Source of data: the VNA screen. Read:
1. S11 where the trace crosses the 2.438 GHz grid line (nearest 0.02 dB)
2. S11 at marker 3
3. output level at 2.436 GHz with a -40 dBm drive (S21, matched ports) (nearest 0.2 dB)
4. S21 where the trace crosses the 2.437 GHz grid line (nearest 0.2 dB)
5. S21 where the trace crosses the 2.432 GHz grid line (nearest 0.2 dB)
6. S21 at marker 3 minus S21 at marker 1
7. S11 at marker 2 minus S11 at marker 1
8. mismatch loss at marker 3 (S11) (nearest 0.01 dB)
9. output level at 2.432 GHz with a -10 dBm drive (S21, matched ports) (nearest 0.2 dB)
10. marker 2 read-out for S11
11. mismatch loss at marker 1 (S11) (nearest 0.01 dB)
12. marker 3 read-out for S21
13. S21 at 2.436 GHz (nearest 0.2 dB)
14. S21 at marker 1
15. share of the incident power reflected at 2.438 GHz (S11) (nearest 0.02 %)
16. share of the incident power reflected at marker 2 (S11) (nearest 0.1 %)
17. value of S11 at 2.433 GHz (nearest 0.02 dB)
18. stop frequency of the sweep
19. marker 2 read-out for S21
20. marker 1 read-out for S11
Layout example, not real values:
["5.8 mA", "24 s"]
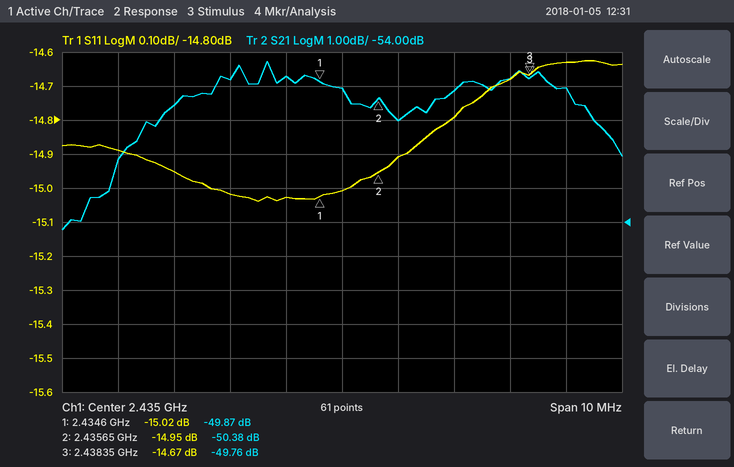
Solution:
["-14.68 dB", "-14.67 dB", "-91.0 dBm", "-50.2 dB", "-50.6 dB", "0.11 dB", "0.07 dB", "0.15 dB", "-60.6 dBm", "-14.95 dB", "0.14 dB", "-49.76 dB", "-51.0 dB", "-49.87 dB", "3.40 %", "3.2 %", "-15.02 dB", "2.44 GHz", "-50.38 dB", "-15.02 dB"]
